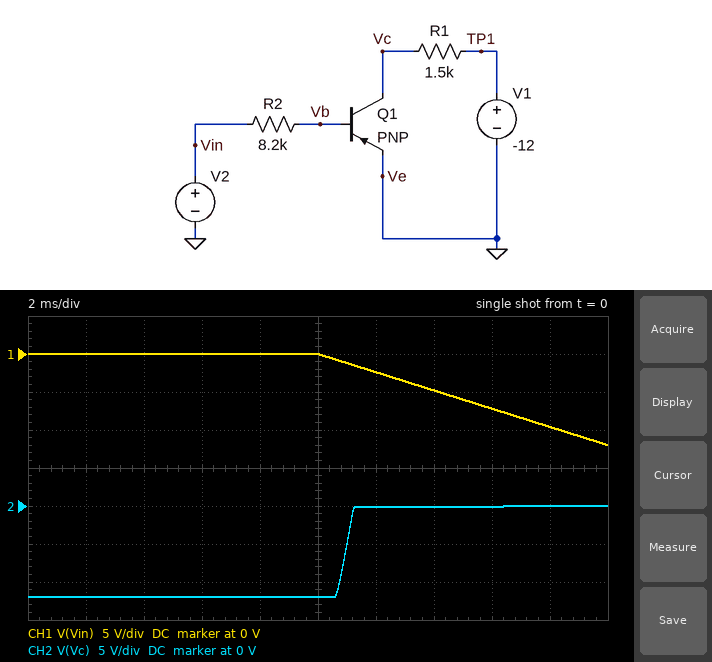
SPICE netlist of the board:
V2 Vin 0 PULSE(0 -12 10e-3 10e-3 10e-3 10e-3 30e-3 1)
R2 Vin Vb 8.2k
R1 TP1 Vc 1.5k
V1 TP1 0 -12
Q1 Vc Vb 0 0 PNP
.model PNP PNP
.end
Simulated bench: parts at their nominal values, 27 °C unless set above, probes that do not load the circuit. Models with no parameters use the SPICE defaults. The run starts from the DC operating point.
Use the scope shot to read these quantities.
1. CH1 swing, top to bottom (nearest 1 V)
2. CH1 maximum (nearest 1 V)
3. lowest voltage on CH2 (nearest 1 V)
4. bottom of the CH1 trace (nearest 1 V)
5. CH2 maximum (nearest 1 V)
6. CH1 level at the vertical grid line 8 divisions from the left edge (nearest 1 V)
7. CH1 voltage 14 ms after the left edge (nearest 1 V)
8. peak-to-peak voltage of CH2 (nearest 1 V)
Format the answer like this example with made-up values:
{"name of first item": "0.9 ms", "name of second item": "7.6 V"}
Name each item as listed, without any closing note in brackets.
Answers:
{"CH1 swing, top to bottom": "12 V", "CH1 maximum": "0 V", "lowest voltage on CH2": "-12 V", "bottom of the CH1 trace": "-12 V", "CH2 maximum": "0 V", "CH1 level at the vertical grid line 8 divisions from the left edge": "-7 V", "CH1 voltage 14 ms after the left edge": "-5 V", "peak-to-peak voltage of CH2": "12 V"}
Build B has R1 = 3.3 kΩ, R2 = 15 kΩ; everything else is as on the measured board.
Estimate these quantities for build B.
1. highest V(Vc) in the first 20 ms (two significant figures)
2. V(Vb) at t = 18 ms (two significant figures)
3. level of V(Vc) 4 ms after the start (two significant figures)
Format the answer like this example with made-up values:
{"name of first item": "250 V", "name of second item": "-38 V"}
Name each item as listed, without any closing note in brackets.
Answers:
{"highest V(Vc) in the first 20 ms": "-51 mV", "V(Vb) at t = 18 ms": "-810 mV", "level of V(Vc) 4 ms after the start": "-12 V"}
